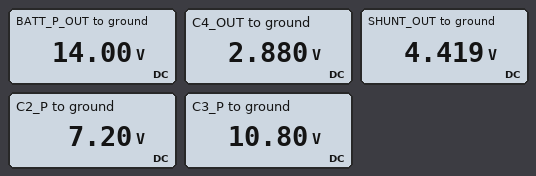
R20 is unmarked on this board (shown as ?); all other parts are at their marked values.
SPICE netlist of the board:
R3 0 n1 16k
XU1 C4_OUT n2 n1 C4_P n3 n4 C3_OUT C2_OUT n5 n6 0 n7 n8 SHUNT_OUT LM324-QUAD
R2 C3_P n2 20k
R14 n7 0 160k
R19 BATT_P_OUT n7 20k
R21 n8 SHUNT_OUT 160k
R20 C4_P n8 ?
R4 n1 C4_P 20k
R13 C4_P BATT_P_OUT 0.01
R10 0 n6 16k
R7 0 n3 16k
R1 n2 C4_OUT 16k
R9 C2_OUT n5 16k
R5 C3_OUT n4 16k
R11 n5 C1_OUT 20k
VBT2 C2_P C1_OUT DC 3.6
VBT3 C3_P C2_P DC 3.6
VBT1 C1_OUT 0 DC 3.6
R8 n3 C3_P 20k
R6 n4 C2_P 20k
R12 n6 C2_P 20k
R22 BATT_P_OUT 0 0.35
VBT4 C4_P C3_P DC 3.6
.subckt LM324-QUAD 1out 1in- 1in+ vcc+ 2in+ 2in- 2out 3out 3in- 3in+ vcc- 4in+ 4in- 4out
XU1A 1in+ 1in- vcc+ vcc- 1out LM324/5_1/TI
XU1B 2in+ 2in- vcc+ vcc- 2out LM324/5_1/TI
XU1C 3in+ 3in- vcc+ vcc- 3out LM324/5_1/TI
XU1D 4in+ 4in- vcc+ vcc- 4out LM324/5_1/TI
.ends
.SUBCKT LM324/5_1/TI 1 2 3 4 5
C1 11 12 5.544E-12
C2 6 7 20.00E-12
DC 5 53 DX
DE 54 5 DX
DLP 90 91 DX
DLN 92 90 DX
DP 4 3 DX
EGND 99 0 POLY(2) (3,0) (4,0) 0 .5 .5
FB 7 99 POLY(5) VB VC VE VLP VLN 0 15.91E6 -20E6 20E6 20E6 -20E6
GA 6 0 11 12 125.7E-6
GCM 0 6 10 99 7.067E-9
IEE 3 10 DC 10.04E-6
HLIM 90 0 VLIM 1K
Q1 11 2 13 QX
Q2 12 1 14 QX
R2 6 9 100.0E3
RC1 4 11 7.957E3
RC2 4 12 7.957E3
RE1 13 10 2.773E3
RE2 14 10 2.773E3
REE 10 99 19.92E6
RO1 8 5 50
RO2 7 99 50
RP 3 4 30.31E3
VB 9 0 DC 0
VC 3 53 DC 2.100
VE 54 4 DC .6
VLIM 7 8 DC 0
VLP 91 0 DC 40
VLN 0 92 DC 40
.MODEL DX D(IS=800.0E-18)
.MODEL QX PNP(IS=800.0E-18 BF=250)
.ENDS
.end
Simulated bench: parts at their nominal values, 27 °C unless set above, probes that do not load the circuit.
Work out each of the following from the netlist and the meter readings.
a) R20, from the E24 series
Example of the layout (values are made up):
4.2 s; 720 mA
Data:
39 kΩ
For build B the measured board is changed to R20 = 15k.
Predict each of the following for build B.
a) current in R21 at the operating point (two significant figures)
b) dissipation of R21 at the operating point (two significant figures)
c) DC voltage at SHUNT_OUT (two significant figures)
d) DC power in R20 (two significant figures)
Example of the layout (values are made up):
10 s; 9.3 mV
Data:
82 µA; 1.1 mW; 5.3 mV; 100 µW
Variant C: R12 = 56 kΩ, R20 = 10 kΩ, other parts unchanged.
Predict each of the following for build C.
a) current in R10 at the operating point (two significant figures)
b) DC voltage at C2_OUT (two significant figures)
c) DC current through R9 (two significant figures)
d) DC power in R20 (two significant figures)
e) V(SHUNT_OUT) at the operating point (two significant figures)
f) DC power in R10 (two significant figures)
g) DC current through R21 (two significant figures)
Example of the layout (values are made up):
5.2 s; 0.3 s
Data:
100 µA; 39 mV; 99 µA; 72 µW; 5.3 mV; 160 µW; 85 µA
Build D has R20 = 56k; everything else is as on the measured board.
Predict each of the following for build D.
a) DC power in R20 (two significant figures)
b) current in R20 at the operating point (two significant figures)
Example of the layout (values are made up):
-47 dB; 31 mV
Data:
68 µW; 35 µA
